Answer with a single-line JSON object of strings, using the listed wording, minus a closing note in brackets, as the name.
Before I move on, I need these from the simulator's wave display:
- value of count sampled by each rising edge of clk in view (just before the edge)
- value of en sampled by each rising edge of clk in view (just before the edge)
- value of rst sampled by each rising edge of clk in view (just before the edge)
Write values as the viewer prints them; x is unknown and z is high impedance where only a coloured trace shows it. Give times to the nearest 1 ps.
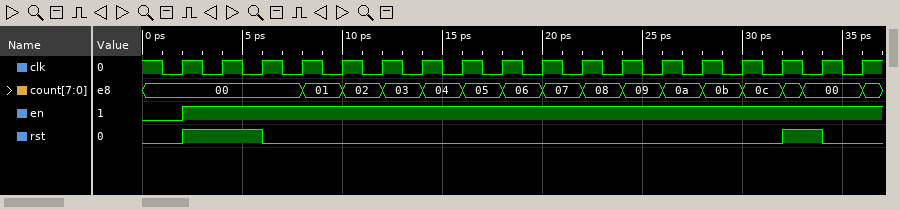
{"value of count sampled by each rising edge of clk in view": "00, 00, 00, 00, 01, 02, 03, 04, 05, 06, 07, 08, 09, 0a, 0b, 0c, 00, 00", "value of en sampled by each rising edge of clk in view": "0 1 1 1 1 1 1 1 1 1 1 1 1 1 1 1 1 1", "value of rst sampled by each rising edge of clk in view": "0 1 1 0 0 0 0 0 0 0 0 0 0 0 0 0 1 0"}
